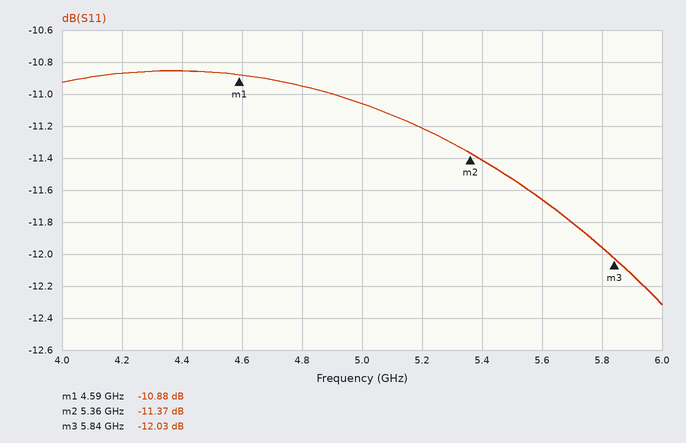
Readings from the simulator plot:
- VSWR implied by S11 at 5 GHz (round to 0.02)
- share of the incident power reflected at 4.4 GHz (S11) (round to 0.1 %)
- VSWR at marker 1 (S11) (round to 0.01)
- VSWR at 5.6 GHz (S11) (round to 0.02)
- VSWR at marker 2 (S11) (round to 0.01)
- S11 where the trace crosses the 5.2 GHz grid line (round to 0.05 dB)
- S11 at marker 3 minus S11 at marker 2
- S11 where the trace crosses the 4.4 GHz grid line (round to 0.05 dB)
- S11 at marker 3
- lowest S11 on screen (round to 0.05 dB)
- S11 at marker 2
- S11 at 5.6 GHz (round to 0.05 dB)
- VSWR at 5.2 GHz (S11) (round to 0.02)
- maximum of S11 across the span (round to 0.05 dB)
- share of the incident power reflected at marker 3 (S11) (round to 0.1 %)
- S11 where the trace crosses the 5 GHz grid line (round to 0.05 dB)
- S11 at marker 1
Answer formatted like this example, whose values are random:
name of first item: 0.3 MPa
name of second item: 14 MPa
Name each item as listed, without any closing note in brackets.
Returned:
VSWR implied by S11 at 5 GHz: 1.78
share of the incident power reflected at 4.4 GHz (S11): 8.2 %
VSWR at marker 1 (S11): 1.80
VSWR at 5.6 GHz (S11): 1.70
VSWR at marker 2 (S11): 1.74
S11 where the trace crosses the 5.2 GHz grid line: -11.20 dB
S11 at marker 3 minus S11 at marker 2: -0.66 dB
S11 where the trace crosses the 4.4 GHz grid line: -10.85 dB
S11 at marker 3: -12.03 dB
lowest S11 on screen: -12.30 dB
S11 at marker 2: -11.37 dB
S11 at 5.6 GHz: -11.65 dB
VSWR at 5.2 GHz (S11): 1.76
maximum of S11 across the span: -10.85 dB
share of the incident power reflected at marker 3 (S11): 6.3 %
S11 where the trace crosses the 5 GHz grid line: -11.05 dB
S11 at marker 1: -10.88 dB
